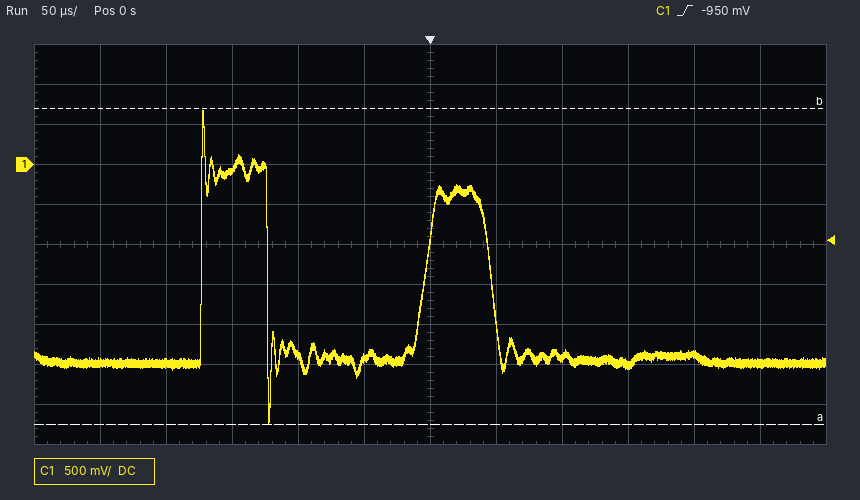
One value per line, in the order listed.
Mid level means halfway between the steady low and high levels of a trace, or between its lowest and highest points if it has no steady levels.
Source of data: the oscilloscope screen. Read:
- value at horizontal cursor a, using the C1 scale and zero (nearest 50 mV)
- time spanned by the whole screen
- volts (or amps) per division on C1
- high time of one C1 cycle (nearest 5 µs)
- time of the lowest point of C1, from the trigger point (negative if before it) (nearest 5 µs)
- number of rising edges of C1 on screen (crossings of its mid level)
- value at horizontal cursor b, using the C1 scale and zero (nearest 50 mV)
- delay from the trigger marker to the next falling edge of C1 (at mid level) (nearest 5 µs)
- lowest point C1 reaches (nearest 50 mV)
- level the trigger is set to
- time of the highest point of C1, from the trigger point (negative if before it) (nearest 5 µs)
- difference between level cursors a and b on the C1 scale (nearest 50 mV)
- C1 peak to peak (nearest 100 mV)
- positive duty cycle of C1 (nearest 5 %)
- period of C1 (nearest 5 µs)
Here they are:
-3.25 V
600 µs
500 mV
50 µs
-120 µs
2
700 mV
45 µs
-3.25 V
-950 mV
-170 µs
3.95 V
3.90 V
30 %
170 µs
